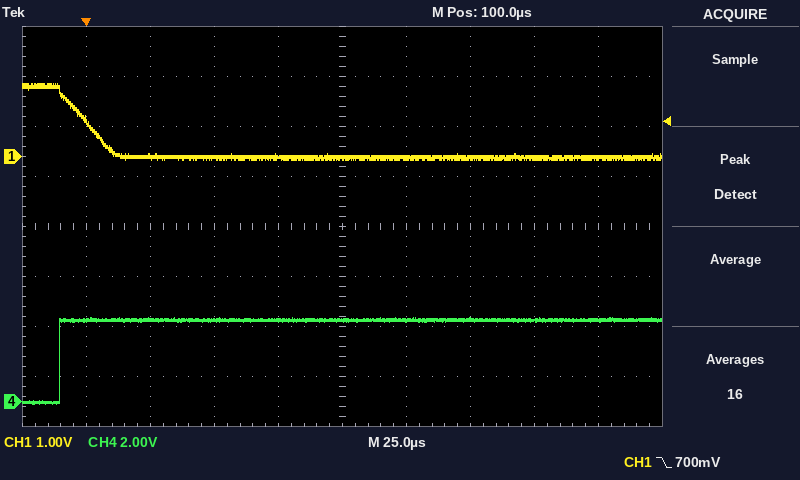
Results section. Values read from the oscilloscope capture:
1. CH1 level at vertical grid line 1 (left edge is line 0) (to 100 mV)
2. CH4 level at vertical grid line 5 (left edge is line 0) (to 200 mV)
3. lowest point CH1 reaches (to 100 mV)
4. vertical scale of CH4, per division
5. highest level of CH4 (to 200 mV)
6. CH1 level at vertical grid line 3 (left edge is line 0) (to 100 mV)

700 mV
3.2 V
-100 mV
2 V
3.4 V
0.0 V
